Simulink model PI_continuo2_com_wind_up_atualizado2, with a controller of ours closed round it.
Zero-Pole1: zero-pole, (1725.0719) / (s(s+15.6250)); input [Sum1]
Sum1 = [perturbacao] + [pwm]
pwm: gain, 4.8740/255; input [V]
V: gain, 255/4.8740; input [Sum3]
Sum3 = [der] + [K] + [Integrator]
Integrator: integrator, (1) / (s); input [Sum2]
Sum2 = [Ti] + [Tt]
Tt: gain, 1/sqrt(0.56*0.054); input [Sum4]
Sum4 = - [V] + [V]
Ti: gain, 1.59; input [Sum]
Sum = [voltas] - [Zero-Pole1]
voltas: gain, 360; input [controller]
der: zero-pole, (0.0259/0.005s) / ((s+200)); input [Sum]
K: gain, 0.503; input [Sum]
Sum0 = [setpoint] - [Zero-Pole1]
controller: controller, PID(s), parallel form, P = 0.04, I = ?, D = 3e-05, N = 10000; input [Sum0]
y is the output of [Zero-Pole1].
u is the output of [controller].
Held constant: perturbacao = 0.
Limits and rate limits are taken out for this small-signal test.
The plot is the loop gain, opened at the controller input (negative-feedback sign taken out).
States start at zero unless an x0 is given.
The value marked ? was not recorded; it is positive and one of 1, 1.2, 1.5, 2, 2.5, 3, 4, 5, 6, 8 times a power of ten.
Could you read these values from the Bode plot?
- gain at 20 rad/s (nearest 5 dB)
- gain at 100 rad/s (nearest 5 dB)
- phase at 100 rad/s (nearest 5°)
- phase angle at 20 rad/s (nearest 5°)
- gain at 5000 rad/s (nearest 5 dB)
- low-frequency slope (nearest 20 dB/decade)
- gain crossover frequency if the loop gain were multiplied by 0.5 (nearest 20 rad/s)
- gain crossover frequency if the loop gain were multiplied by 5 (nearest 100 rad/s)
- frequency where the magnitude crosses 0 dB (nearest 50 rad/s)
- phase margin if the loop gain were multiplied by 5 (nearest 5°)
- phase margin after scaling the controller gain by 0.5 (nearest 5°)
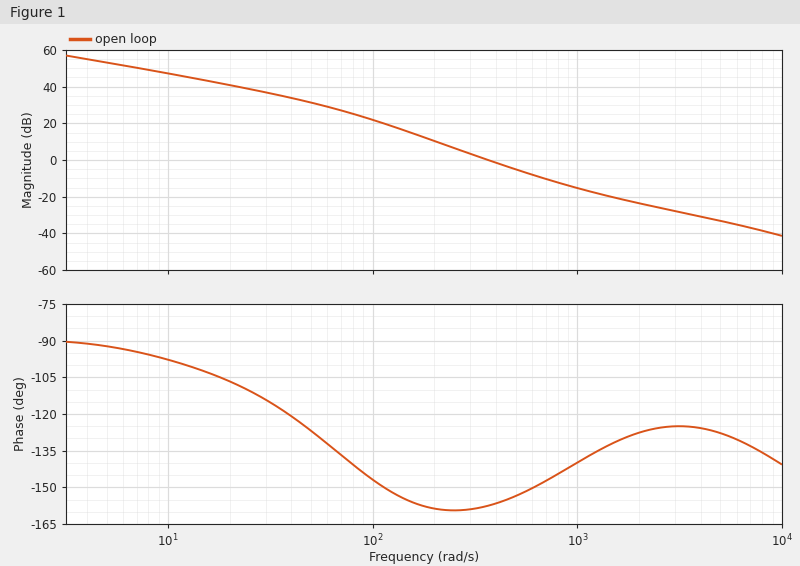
40 dB
20 dB
-145°
-105°
-35 dB
-20 dB/decade
260 rad/s
900 rad/s
350 rad/s
40°
20°
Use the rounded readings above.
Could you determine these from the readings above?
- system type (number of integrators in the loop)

1
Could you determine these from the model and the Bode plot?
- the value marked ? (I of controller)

6
